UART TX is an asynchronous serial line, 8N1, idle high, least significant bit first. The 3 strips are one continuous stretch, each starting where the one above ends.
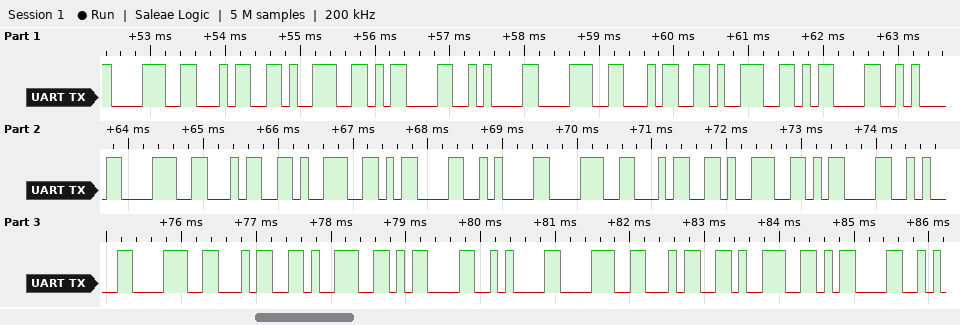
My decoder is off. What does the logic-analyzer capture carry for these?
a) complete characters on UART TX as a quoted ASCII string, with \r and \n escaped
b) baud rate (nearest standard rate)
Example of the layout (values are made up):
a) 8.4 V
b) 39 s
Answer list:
a) "849\r\n849\r\n849\r\n849\r\n849\r\n849\r"
b) 9600 baud
